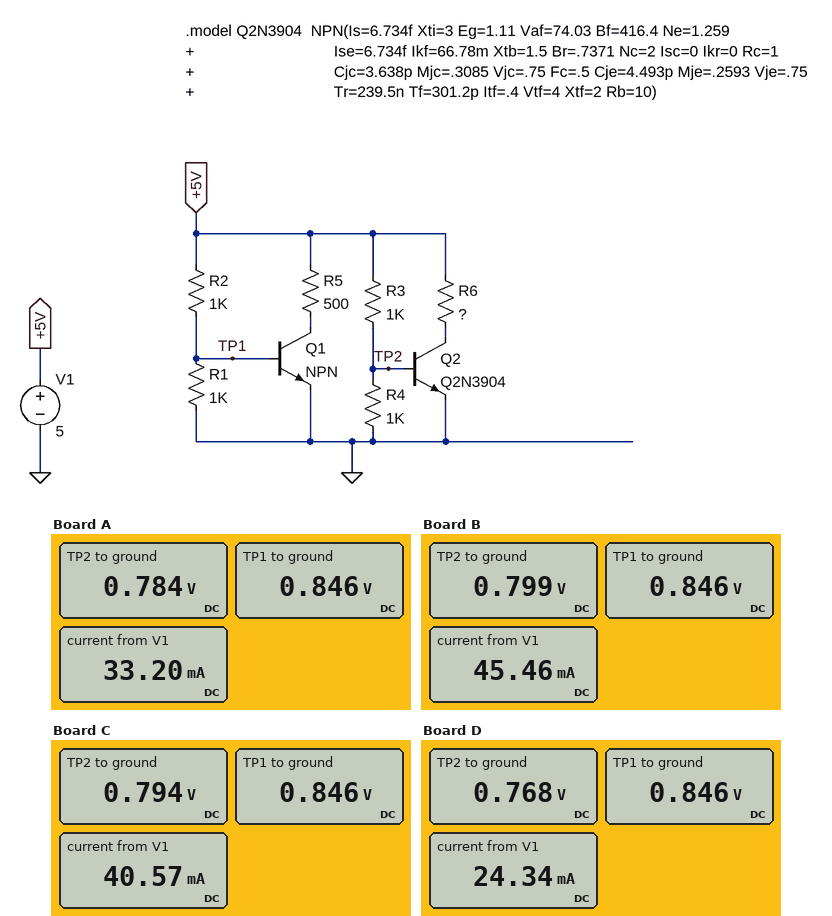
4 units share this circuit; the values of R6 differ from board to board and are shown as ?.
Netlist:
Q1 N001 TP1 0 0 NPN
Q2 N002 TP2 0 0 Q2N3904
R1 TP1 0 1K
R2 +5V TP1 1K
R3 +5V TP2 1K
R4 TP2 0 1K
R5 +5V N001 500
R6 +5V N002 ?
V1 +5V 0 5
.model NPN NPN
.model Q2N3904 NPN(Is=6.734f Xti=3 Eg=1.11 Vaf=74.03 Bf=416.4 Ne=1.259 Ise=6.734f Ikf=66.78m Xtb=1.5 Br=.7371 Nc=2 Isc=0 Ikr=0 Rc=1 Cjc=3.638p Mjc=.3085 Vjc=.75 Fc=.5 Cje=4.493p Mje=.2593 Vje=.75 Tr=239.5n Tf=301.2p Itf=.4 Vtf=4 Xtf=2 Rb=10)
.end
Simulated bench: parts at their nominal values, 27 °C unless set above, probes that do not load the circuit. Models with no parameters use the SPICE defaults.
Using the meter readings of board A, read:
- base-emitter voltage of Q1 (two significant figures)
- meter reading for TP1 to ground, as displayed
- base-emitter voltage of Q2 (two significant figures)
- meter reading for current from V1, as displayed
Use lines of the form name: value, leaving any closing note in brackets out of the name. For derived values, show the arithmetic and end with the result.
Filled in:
base-emitter voltage of Q1: 846 mV = 850 mV
meter reading for TP1 to ground, as displayed: 0.846 V
base-emitter voltage of Q2: 784 mV = 780 mV
meter reading for current from V1, as displayed: 33.20 mA
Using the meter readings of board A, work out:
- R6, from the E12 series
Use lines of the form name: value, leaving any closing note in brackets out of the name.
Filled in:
R6, from the E12 series: 330 Ω
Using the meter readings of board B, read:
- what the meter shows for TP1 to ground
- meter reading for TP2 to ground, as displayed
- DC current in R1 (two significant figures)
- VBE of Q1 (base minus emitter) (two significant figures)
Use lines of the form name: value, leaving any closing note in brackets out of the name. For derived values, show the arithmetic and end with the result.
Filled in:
what the meter shows for TP1 to ground: 0.846 V
meter reading for TP2 to ground, as displayed: 0.799 V
DC current in R1: (846 mV) / 1 kΩ = 850 µA
VBE of Q1 (base minus emitter): 846 mV = 850 mV
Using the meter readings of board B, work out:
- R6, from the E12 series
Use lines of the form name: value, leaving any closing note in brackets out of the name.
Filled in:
R6, from the E12 series: 180 Ω
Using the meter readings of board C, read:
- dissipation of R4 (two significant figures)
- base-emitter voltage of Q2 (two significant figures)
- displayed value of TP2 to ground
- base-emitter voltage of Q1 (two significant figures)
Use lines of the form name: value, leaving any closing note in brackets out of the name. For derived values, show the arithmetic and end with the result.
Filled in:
dissipation of R4: (794 mV)^2 / 1 kΩ = 630 µW
base-emitter voltage of Q2: 794 mV = 790 mV
displayed value of TP2 to ground: 0.794 V
base-emitter voltage of Q1: 846 mV = 850 mV
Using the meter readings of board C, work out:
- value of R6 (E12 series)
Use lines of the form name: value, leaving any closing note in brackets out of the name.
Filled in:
value of R6: 220 Ω
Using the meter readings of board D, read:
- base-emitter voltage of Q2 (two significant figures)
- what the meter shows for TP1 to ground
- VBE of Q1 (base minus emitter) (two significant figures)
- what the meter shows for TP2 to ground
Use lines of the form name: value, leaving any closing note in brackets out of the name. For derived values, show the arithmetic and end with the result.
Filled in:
base-emitter voltage of Q2: 768 mV = 770 mV
what the meter shows for TP1 to ground: 0.846 V
VBE of Q1 (base minus emitter): 846 mV = 850 mV
what the meter shows for TP2 to ground: 0.768 V
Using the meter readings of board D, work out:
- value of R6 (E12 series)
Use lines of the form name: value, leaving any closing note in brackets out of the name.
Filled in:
value of R6: 820 Ω
